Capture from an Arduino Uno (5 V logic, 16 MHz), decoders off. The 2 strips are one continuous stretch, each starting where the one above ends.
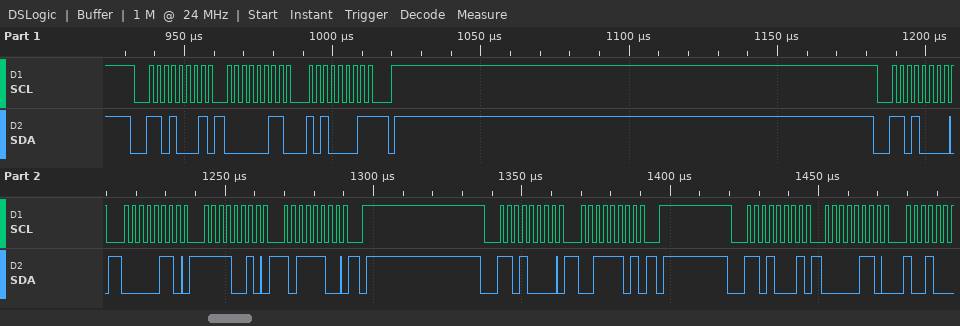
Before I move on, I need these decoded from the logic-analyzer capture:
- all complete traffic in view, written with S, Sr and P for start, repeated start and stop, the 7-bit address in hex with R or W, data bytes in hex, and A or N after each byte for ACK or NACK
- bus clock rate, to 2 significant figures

S 68R A 03 A A1 N P S 68W A 06 A F2 A BC A P S 68W A 3D A P S 68R A 06 A
400 kHz
